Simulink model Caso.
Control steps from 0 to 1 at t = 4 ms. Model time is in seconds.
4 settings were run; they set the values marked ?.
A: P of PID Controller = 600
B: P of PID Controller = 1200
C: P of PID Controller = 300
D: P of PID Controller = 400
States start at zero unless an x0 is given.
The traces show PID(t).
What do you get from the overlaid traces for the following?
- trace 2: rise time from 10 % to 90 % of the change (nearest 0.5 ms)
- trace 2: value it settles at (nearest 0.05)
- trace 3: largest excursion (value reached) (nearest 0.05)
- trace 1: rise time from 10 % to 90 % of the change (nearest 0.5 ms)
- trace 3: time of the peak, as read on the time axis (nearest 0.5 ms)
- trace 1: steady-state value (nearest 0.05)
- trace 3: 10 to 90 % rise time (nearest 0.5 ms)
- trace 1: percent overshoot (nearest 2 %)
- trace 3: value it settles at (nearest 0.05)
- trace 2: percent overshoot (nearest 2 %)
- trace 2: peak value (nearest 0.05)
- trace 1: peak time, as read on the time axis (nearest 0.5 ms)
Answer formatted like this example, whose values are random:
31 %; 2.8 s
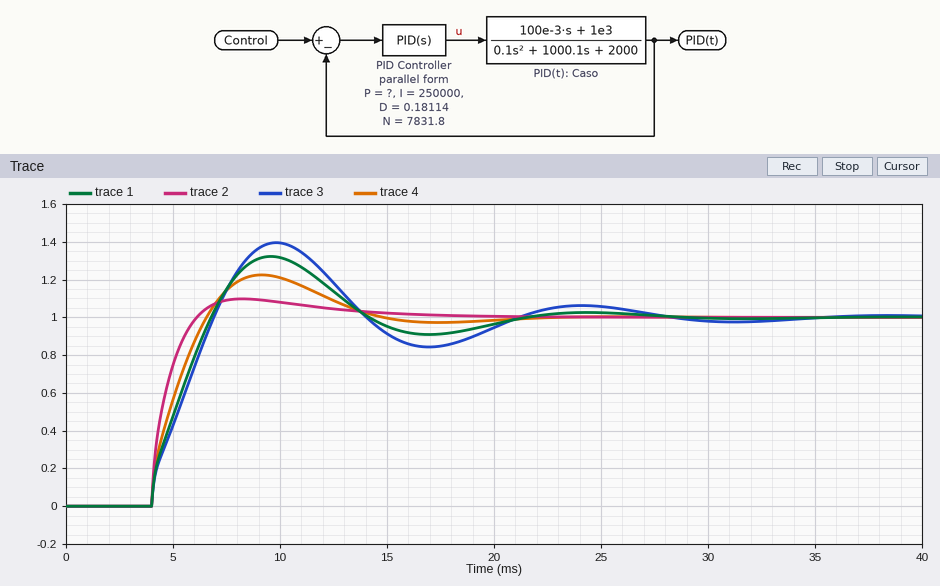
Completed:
1.5 ms; 1.00; 1.40; 2.5 ms; 10.0 ms; 1.00; 2.5 ms; 32 %; 1.00; 10 %; 1.10; 9.5 ms
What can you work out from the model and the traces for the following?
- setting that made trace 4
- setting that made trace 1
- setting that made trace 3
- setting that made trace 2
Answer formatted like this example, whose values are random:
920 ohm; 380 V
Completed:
A; D; C; B
